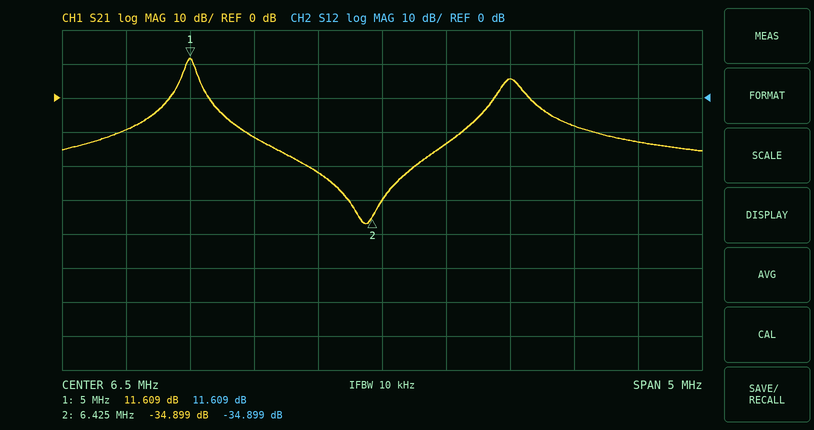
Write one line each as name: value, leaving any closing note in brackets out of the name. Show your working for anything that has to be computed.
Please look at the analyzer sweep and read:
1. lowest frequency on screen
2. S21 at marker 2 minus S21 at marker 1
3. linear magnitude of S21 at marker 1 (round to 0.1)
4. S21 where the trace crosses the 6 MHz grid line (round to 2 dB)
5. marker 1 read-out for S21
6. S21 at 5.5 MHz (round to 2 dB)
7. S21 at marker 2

lowest frequency on screen: 4 MHz
S21 at marker 2 minus S21 at marker 1: -34.899 − (11.609) = -46.508 dB
linear magnitude of S21 at marker 1: 10^(11.609/20) ≈ 3.8
S21 where the trace crosses the 6 MHz grid line: -22 dB
marker 1 read-out for S21: 11.609 dB
S21 at 5.5 MHz: -12 dB
S21 at marker 2: -34.899 dB
